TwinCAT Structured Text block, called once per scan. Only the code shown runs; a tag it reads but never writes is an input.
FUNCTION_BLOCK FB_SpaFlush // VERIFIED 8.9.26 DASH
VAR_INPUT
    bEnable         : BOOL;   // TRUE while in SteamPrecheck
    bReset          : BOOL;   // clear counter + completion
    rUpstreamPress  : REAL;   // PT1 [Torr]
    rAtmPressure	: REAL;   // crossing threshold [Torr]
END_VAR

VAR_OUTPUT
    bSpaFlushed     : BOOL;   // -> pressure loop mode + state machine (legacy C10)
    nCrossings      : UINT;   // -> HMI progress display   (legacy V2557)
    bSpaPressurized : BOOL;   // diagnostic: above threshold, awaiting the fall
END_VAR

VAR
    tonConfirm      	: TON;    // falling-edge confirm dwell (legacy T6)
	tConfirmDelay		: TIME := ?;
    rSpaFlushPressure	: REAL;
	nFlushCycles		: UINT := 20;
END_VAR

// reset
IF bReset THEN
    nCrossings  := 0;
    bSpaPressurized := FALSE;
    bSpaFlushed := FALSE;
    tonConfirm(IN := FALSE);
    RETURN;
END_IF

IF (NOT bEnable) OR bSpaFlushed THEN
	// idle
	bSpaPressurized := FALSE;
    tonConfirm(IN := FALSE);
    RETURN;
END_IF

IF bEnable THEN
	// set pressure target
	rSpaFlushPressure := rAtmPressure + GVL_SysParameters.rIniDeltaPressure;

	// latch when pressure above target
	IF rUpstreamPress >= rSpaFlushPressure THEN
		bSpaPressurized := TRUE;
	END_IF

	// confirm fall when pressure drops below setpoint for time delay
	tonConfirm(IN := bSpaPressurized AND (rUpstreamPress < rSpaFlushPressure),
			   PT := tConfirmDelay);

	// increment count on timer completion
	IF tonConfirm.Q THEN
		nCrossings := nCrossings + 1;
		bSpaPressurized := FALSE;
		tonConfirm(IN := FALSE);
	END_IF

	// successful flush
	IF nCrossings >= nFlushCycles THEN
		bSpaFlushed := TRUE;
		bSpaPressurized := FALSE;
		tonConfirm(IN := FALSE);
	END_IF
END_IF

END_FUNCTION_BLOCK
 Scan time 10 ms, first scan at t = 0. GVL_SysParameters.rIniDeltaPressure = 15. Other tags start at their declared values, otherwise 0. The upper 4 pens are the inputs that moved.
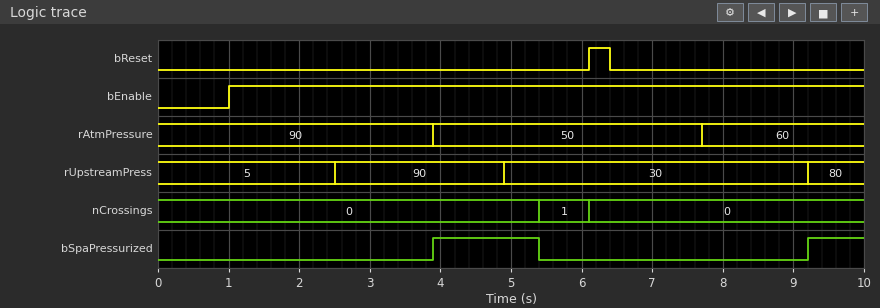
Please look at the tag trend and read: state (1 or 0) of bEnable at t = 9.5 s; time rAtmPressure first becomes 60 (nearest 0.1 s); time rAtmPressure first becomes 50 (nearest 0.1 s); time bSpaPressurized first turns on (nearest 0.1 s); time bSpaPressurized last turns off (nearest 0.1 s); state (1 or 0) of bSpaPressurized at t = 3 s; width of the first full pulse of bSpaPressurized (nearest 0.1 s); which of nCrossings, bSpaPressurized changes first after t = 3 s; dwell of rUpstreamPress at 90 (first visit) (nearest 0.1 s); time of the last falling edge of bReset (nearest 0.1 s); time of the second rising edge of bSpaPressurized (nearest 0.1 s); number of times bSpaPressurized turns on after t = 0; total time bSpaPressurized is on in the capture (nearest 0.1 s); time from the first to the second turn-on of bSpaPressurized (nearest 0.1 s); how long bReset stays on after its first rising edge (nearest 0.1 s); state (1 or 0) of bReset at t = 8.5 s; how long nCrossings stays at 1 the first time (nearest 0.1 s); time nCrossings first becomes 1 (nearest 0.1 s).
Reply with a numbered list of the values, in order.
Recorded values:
1. 1
2. 7.7 s
3. 3.9 s
4. 3.9 s
5. 5.4 s
6. 0
7. 1.5 s
8. bSpaPressurized
9. 2.4 s
10. 6.4 s
11. 9.2 s
12. 2
13. 2.3 s
14. 5.3 s
15. 0.3 s
16. 0
17. 0.7 s
18. 5.4 s
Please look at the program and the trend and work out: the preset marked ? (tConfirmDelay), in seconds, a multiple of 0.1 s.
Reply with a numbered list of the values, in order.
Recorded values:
1. 0.5 s
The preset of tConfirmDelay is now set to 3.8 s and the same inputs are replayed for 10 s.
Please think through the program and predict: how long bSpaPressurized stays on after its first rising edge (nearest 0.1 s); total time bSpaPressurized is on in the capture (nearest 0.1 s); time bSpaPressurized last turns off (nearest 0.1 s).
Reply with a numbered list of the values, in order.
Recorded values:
1. 2.2 s
2. 3.0 s
3. 6.1 s
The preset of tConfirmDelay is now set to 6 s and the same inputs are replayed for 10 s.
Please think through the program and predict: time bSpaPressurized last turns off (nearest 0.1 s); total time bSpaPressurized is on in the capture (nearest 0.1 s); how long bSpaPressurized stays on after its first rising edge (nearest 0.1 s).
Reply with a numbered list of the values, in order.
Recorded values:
1. 6.1 s
2. 3.0 s
3. 2.2 s
